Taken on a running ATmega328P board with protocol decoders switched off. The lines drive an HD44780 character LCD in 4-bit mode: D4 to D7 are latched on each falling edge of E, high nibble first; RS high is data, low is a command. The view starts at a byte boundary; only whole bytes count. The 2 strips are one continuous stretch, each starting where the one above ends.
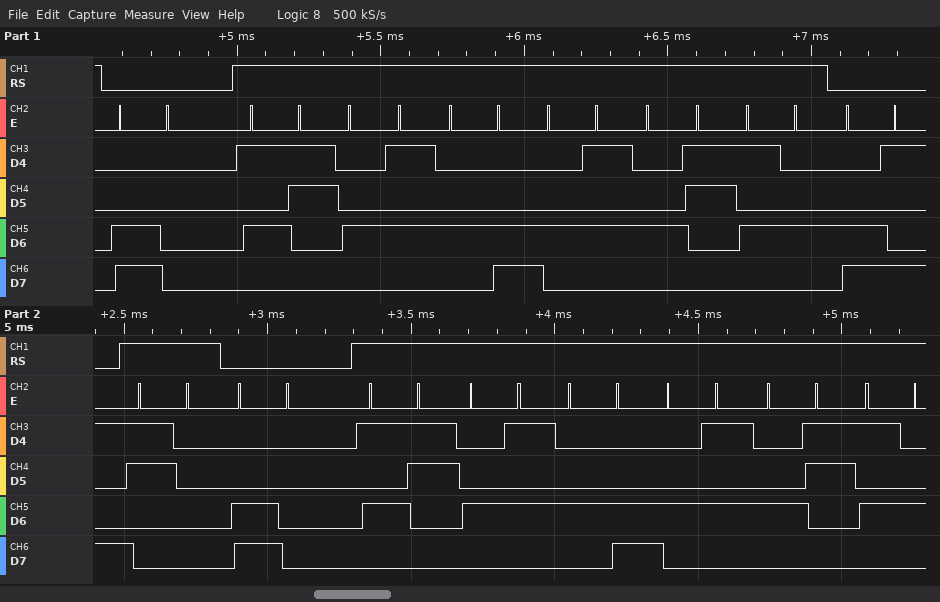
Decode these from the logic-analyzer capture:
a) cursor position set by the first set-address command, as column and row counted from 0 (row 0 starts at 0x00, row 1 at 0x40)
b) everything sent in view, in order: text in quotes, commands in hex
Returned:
column 0, row 1
0xC0 "SELECT" 0xC9 "0" 0xC0 "SELECT"
